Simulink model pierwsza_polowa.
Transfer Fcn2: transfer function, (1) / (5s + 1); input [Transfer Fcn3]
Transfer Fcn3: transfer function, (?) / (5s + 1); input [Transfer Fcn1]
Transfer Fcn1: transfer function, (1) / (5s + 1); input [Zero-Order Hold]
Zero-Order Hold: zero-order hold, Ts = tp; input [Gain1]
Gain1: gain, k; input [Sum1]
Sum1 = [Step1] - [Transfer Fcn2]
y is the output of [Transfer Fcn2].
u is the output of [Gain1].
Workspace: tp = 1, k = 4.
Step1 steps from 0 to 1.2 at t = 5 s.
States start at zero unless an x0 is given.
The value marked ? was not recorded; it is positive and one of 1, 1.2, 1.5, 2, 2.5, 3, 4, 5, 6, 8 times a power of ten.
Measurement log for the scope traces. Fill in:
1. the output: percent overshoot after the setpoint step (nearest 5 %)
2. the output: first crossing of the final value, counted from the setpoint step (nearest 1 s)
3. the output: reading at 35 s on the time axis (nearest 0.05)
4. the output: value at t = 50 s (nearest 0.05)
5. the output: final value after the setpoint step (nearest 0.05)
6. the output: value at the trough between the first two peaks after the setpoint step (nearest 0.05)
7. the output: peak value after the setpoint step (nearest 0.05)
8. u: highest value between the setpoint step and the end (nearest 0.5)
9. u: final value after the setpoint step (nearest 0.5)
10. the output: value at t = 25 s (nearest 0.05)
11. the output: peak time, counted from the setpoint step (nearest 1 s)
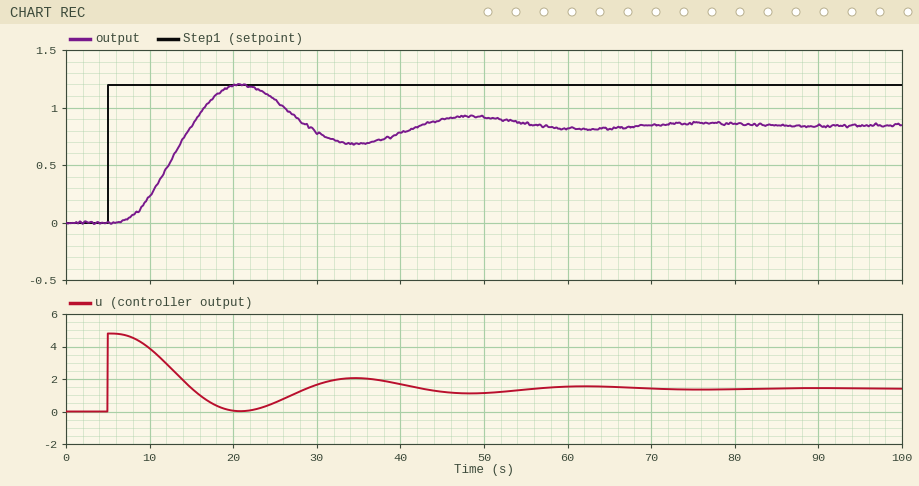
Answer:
40 %
10 s
0.70
0.90
0.85
0.70
1.20
5.0
1.5
1.05
16 s
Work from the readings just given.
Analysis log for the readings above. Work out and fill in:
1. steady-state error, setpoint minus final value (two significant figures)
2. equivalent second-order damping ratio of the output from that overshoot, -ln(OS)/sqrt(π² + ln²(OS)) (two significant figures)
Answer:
0.35
0.28
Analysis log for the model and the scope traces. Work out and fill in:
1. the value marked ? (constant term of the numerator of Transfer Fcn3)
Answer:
0.6
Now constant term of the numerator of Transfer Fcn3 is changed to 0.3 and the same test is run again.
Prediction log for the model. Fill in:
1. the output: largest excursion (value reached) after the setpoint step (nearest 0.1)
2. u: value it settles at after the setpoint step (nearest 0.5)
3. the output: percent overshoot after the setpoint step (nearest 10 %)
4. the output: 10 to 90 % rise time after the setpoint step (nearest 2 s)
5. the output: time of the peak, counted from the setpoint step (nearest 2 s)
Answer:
0.8
2.0
20 %
8 s
20 s
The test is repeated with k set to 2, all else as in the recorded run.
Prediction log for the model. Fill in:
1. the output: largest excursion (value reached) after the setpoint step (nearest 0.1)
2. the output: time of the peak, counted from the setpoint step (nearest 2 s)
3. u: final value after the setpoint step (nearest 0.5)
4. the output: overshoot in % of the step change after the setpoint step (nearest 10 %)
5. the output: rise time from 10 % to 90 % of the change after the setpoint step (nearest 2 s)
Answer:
0.8
20 s
1.0
20 %
8 s
